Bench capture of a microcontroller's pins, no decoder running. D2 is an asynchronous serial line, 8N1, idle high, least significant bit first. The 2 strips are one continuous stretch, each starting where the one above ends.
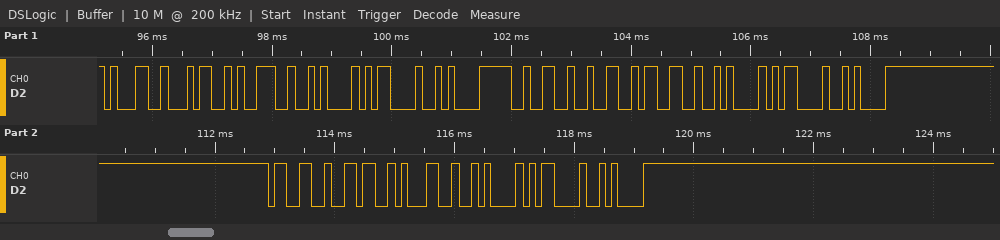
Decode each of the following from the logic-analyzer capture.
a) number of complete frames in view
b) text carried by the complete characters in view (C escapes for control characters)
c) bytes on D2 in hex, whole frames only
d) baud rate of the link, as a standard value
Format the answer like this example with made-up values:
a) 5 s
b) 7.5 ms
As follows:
a) 18
b) "149\n\r\n223\n\r\n361\n\r\n"
c) 31 34 39 0A 0D 0A 32 32 33 0A 0D 0A 33 36 31 0A 0D 0A
d) 9600 baud
